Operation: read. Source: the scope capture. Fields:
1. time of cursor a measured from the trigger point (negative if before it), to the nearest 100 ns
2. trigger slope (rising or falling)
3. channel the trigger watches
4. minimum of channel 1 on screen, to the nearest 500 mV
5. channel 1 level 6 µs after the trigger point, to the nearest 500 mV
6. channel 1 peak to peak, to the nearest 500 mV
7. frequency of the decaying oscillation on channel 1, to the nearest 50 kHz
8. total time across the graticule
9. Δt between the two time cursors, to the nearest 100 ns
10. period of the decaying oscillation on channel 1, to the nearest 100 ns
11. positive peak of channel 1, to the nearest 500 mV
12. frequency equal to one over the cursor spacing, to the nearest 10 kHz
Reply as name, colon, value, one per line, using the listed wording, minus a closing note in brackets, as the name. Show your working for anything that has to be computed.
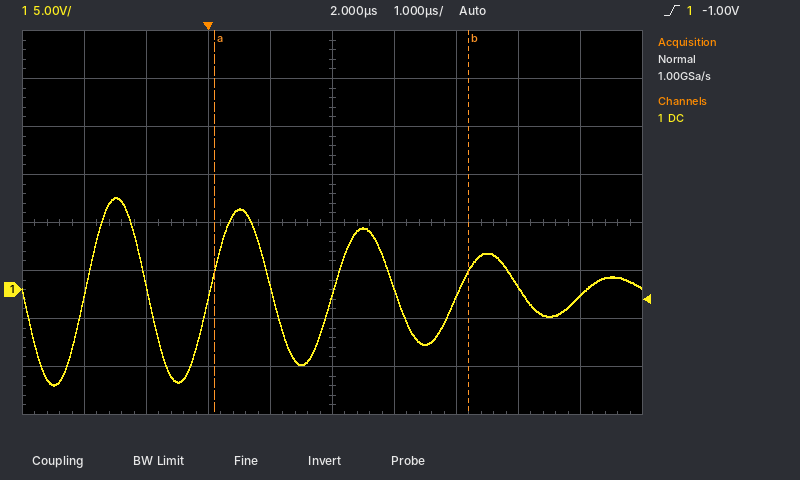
time of cursor a measured from the trigger point (negative if before it), to the nearest 100 ns: +100 ns
trigger slope: rising
channel the trigger watches: channel 1
minimum of channel 1 on screen, to the nearest 500 mV: -10.0 V
channel 1 level 6 µs after the trigger point, to the nearest 500 mV: -500 mV
channel 1 peak to peak, to the nearest 500 mV: 9.5 V − (-10.0 V) = 19.5 V
frequency of the decaying oscillation on channel 1, to the nearest 50 kHz: 1 / 2.0 µs ≈ 500 kHz
total time across the graticule: 10 µs
Δt between the two time cursors, to the nearest 100 ns: 4.1 µs
period of the decaying oscillation on channel 1, to the nearest 100 ns: 2.0 µs
positive peak of channel 1, to the nearest 500 mV: 9.5 V
frequency equal to one over the cursor spacing, to the nearest 10 kHz: 1 / 4.1 µs ≈ 240 kHz
